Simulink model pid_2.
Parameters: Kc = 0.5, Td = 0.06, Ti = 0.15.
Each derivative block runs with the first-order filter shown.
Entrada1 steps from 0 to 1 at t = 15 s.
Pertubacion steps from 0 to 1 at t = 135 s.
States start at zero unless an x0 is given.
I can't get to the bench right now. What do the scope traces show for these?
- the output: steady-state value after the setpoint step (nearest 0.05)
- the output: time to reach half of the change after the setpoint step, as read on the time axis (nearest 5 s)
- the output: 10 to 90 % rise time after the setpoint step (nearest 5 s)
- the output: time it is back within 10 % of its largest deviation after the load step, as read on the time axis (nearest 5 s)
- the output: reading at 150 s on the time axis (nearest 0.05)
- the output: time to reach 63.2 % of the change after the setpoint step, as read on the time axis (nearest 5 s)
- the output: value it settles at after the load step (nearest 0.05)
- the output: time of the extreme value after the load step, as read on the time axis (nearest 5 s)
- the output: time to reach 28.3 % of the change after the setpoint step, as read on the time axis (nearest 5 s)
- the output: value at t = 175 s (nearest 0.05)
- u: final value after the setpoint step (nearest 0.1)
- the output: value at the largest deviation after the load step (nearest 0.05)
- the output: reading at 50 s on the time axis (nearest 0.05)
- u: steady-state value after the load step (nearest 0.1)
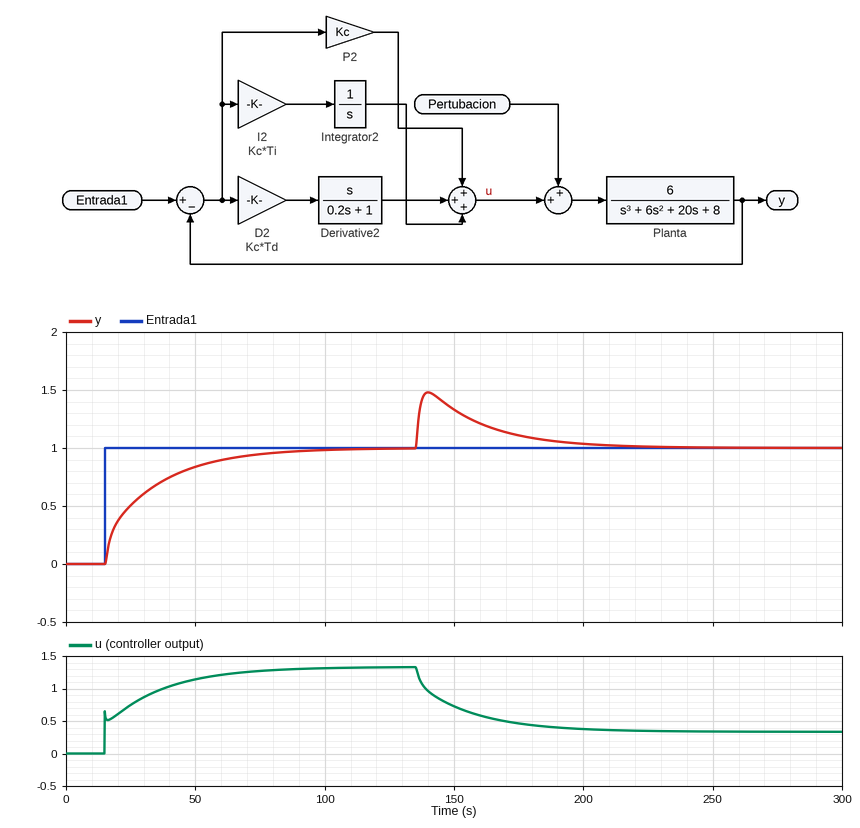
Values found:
1.00
25 s
45 s
195 s
1.35
30 s
1.00
140 s
20 s
1.10
1.3
1.50
0.85
0.3
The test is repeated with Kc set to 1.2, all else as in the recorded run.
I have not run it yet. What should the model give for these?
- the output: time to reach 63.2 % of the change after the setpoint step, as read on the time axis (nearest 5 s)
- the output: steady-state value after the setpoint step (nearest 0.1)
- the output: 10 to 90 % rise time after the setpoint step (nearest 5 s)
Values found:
20 s
1.0
20 s
